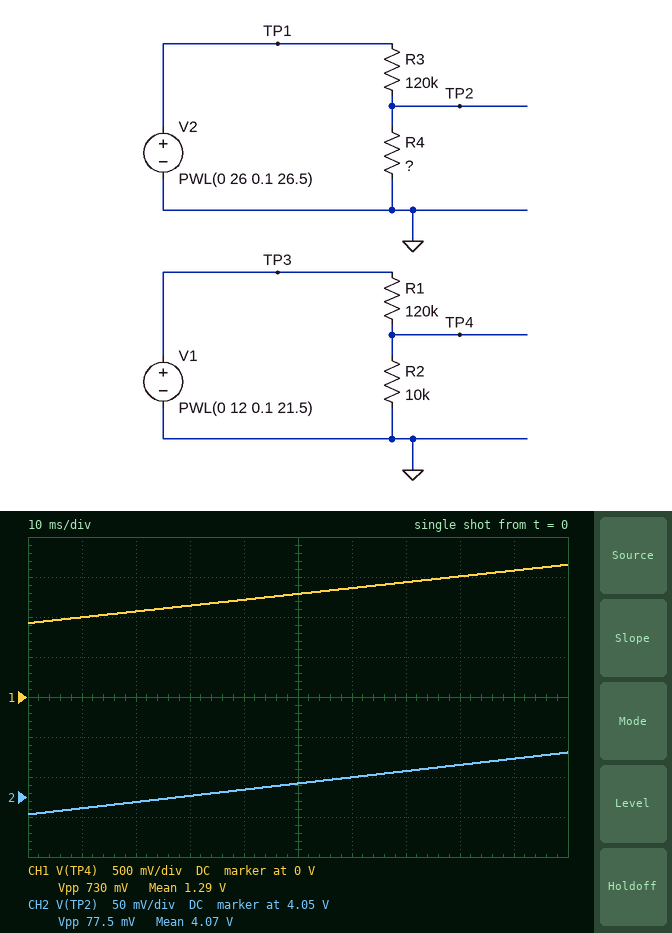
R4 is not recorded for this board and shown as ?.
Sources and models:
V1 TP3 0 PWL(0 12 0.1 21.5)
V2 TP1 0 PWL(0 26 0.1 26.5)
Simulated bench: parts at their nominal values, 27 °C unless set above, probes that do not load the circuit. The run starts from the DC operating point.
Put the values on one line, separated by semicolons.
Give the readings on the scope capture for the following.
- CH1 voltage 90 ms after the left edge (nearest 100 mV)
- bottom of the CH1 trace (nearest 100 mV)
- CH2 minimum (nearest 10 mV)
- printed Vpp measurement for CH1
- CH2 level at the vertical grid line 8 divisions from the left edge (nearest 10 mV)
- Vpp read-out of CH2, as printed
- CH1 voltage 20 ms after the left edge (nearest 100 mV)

1.6 V; 900 mV; 4.03 V; 730 mV; 4.09 V; 77.5 mV; 1.1 V
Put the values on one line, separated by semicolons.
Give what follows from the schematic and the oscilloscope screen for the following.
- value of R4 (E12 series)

22 kΩ
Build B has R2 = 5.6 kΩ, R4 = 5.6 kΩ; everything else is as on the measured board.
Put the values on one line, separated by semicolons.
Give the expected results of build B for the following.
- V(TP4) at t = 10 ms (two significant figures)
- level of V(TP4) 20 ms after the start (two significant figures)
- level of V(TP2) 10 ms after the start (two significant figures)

580 mV; 620 mV; 1.2 V
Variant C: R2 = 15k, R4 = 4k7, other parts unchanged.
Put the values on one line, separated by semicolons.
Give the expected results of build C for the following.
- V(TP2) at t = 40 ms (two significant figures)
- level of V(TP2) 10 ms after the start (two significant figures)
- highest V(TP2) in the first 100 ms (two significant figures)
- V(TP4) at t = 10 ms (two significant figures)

990 mV; 980 mV; 1.0 V; 1.4 V
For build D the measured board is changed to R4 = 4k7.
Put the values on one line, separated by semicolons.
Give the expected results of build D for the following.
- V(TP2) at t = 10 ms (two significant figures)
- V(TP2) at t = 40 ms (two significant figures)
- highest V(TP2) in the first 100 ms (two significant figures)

980 mV; 990 mV; 1.0 V
